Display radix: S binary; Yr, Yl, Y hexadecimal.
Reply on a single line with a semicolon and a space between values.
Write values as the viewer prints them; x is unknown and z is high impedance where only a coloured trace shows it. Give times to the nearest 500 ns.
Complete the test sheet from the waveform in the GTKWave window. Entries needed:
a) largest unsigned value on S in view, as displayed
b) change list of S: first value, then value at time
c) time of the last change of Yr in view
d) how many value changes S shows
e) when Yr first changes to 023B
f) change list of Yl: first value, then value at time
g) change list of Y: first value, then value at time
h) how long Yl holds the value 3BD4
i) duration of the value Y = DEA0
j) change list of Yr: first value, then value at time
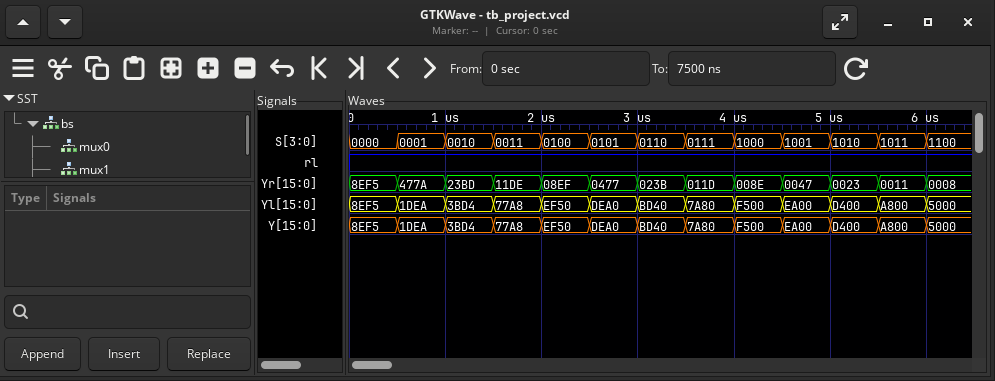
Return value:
1100; 0000, 0001 at 500 ns, 0010 at 1000 ns, 0011 at 1500 ns, 0100 at 2000 ns, 0101 at 2500 ns, 0110 at 3000 ns, 0111 at 3500 ns, 1000 at 4000 ns, 1001 at 4500 ns, 1010 at 5000 ns, 1011 at 5500 ns, 1100 at 6000 ns; 6000 ns; 12; 3000 ns; 8EF5, 1DEA at 500 ns, 3BD4 at 1000 ns, 77A8 at 1500 ns, EF50 at 2000 ns, DEA0 at 2500 ns, BD40 at 3000 ns, 7A80 at 3500 ns, F500 at 4000 ns, EA00 at 4500 ns, D400 at 5000 ns, A800 at 5500 ns, 5000 at 6000 ns; 8EF5, 1DEA at 500 ns, 3BD4 at 1000 ns, 77A8 at 1500 ns, EF50 at 2000 ns, DEA0 at 2500 ns, BD40 at 3000 ns, 7A80 at 3500 ns, F500 at 4000 ns, EA00 at 4500 ns, D400 at 5000 ns, A800 at 5500 ns, 5000 at 6000 ns; 500 ns; 500 ns; 8EF5, 477A at 500 ns, 23BD at 1000 ns, 11DE at 1500 ns, 08EF at 2000 ns, 0477 at 2500 ns, 023B at 3000 ns, 011D at 3500 ns, 008E at 4000 ns, 0047 at 4500 ns, 0023 at 5000 ns, 0011 at 5500 ns, 0008 at 6000 ns
